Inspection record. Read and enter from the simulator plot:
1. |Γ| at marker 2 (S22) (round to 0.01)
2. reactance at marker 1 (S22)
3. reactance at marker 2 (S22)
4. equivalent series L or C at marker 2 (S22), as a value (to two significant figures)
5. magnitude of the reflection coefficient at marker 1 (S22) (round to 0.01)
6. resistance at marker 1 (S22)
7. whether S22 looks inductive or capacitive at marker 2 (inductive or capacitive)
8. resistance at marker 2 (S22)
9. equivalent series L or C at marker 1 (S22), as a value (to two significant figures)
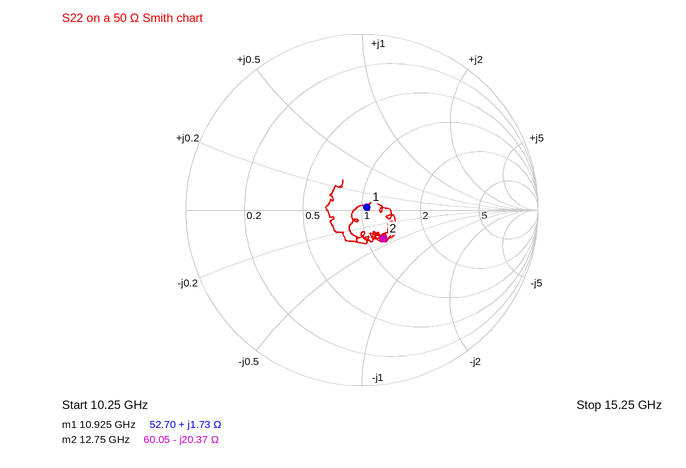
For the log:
0.20
+1.73 Ω
-20.37 Ω
610 fF
0.03
52.70 Ω
capacitive
60.05 Ω
25 pH
